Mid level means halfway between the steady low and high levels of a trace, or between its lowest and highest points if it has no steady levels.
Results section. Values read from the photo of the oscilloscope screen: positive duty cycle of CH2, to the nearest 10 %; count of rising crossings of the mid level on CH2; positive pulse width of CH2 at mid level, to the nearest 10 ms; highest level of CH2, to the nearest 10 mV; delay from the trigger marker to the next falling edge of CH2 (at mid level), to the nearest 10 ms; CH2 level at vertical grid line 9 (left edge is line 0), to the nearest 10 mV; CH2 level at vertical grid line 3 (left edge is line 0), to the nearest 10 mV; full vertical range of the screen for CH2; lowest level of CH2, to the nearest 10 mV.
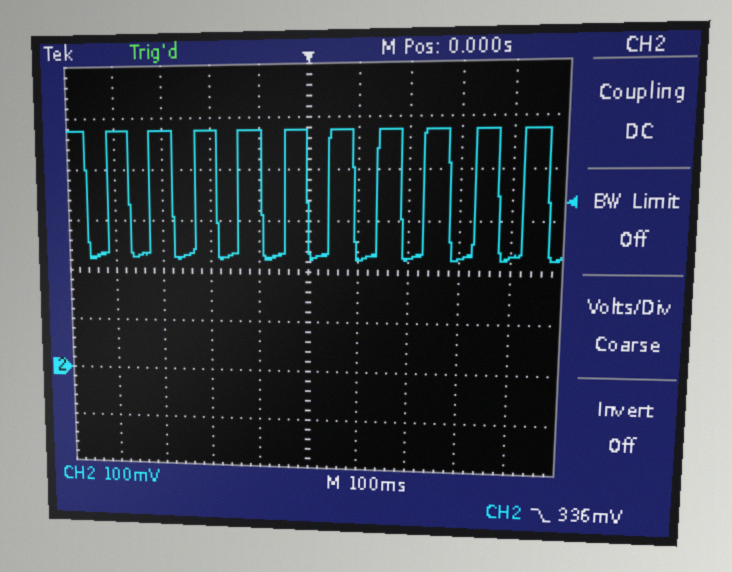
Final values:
50 %
10
50 ms
480 mV
90 ms
230 mV
480 mV
800 mV
220 mV
